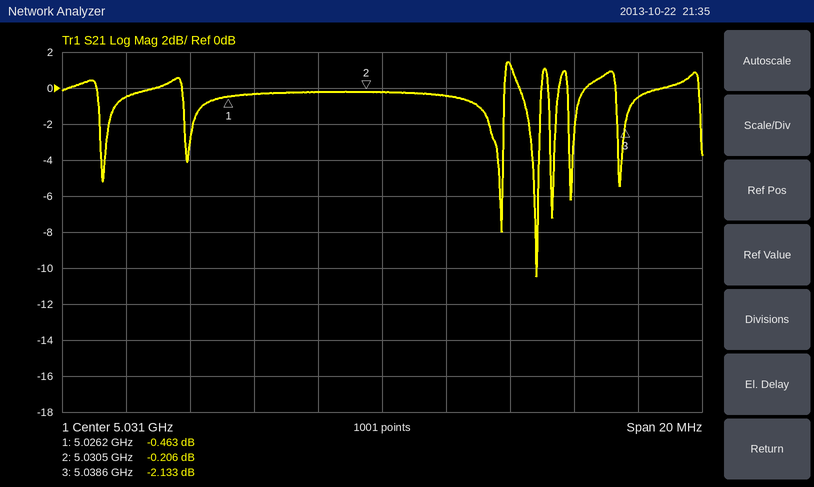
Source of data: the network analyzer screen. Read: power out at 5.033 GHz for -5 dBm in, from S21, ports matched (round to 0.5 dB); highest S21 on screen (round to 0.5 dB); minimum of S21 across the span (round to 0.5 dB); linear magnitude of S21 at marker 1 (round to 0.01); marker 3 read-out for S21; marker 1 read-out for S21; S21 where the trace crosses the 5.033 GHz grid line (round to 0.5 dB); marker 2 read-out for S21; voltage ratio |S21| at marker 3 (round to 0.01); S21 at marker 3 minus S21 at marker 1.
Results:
-5.5 dBm
1.5 dB
-10.5 dB
0.95
-2.133 dB
-0.463 dB
-0.5 dB
-0.206 dB
0.78
-1.670 dB
